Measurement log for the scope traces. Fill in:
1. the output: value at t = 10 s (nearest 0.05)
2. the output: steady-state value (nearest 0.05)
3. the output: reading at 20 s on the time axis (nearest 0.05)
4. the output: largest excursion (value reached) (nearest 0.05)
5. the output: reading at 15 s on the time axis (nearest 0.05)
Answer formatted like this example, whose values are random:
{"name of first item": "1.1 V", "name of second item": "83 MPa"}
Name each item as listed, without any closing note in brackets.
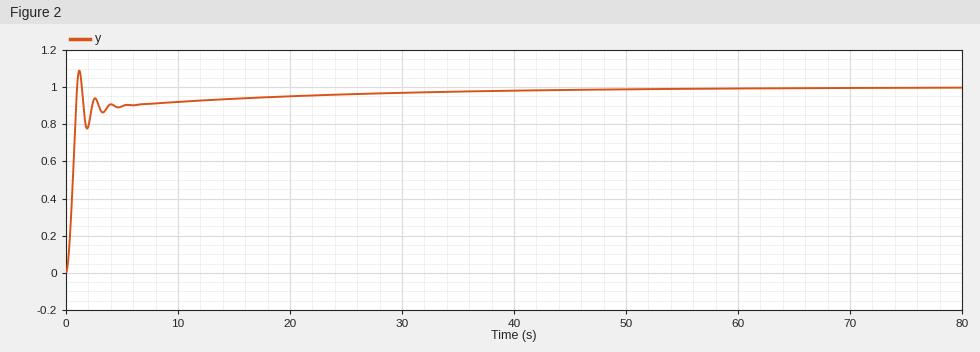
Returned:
{"the output: value at t = 10 s": "0.90", "the output: steady-state value": "1.00", "the output: reading at 20 s on the time axis": "0.95", "the output: largest excursion (value reached)": "1.10", "the output: reading at 15 s on the time axis": "0.95"}
